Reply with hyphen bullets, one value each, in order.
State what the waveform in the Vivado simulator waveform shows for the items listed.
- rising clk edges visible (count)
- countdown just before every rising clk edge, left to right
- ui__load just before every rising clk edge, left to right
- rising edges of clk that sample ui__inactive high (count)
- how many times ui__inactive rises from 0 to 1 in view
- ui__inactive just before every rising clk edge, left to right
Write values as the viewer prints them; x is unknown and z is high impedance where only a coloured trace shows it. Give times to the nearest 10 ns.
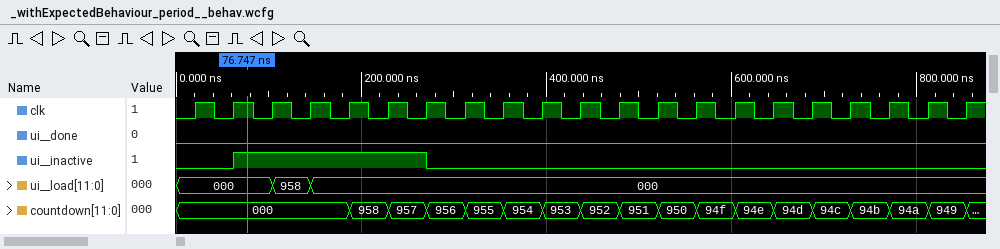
- 21
- 000, 000, 000, 000, 000, 958, 957, 956, 955, 954, 953, 952, 951, 950, 94f, 94e, 94d, 94c, 94b, 94a, 949
- 000, 000, 000, 958, 000, 000, 000, 000, 000, 000, 000, 000, 000, 000, 000, 000, 000, 000, 000, 000, 000
- 5
- 1
- 0 0 1 1 1 1 1 0 0 0 0 0 0 0 0 0 0 0 0 0 0
